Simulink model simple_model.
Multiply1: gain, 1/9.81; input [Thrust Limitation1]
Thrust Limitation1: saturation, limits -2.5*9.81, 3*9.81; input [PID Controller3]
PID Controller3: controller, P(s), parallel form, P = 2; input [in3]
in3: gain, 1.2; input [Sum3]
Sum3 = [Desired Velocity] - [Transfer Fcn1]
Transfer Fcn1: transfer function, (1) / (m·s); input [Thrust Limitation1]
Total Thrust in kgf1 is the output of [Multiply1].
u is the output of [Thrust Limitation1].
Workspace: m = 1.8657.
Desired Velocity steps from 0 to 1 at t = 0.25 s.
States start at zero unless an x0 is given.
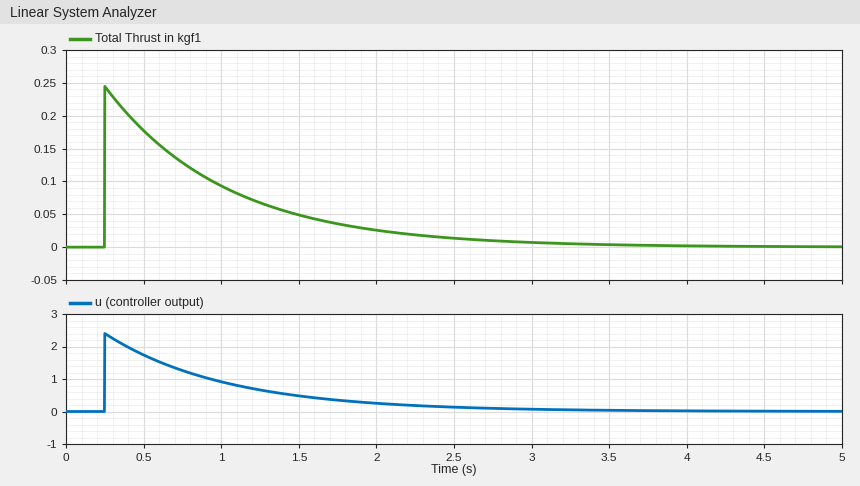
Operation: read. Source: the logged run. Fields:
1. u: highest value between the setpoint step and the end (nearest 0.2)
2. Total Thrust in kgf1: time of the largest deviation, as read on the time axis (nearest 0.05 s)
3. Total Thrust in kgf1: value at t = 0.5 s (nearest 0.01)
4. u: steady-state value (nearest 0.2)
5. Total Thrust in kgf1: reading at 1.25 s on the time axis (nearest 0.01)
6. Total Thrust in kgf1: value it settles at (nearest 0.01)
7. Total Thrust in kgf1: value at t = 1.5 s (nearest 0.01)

2.4
0.25 s
0.18
0.0
0.07
0.00
0.05
